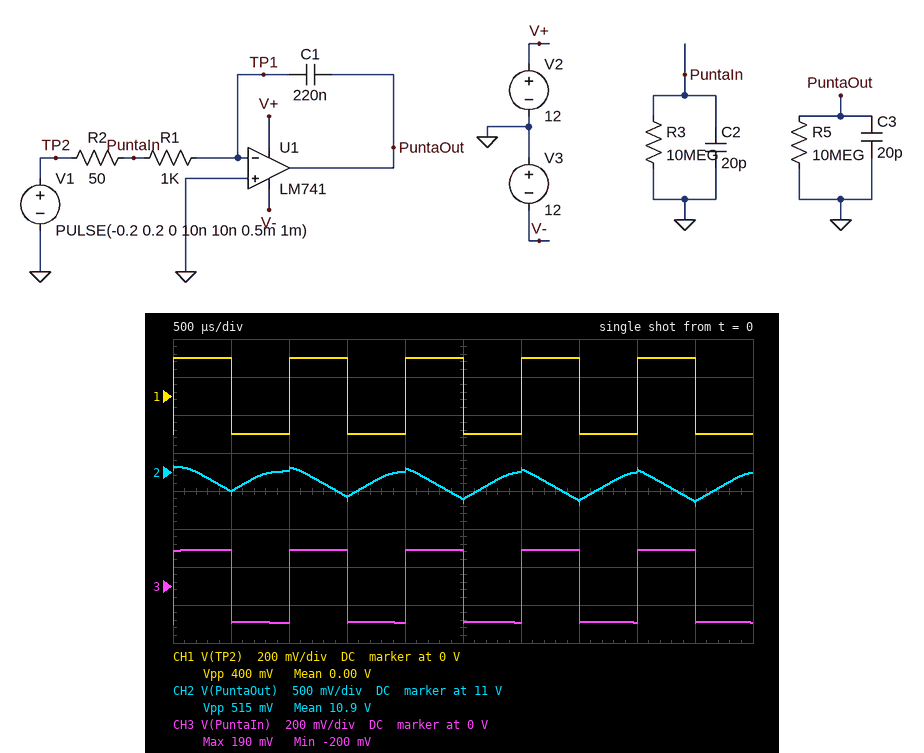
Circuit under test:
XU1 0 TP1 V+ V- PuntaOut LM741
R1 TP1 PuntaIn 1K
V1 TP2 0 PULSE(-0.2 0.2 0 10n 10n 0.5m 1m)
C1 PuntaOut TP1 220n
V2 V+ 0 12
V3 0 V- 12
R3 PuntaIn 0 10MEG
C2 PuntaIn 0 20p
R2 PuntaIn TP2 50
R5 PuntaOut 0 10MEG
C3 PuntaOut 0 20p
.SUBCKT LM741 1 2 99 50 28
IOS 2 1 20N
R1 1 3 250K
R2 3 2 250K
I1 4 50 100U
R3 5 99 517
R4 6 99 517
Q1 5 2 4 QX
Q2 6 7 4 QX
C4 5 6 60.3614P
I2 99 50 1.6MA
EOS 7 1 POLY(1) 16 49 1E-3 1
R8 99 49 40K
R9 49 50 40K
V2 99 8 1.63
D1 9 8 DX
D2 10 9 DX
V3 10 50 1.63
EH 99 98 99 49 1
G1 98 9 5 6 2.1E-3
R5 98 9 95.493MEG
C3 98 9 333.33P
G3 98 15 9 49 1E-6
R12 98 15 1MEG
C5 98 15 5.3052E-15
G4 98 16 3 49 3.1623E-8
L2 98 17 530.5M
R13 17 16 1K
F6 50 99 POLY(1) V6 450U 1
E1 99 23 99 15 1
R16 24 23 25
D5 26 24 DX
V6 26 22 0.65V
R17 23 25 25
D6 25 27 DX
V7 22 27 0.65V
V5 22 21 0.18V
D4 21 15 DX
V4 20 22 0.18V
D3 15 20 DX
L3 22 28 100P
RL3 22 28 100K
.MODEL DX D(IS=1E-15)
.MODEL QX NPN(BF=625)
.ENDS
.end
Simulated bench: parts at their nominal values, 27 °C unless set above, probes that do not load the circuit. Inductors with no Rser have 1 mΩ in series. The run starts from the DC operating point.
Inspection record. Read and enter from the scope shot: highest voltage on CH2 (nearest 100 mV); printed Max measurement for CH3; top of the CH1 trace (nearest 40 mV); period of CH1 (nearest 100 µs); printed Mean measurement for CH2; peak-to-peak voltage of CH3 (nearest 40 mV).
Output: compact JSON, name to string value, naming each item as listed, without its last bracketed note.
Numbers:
{"highest voltage on CH2": "11.1 V", "printed Max measurement for CH3": "190 mV", "top of the CH1 trace": "200 mV", "period of CH1": "1.0 ms", "printed Mean measurement for CH2": "10.9 V", "peak-to-peak voltage of CH3": "400 mV"}
